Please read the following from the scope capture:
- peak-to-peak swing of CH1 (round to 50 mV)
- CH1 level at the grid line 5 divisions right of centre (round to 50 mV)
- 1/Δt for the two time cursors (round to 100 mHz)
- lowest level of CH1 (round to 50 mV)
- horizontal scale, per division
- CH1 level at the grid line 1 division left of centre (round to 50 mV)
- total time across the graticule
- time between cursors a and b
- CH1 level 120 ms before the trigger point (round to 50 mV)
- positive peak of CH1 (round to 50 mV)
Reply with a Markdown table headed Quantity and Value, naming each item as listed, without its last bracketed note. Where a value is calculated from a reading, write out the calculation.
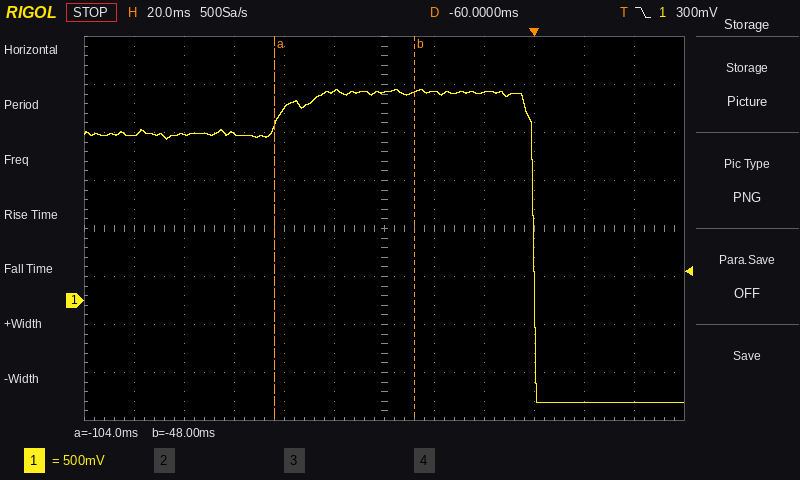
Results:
| Quantity | Value |
|---|---|
| peak-to-peak swing of CH1 | 2.20 V − (-1.05 V) = 3.25 V |
| CH1 level at the grid line 5 divisions right of centre | -1.05 V |
| 1/Δt for the two time cursors | 1 / 56 ms ≈ 17.9 Hz |
| lowest level of CH1 | -1.05 V |
| horizontal scale, per division | 20 ms |
| CH1 level at the grid line 1 division left of centre | 2.20 V |
| total time across the graticule | 240 ms |
| time between cursors a and b | -48 ms − (-104 ms) = 56 ms |
| CH1 level 120 ms before the trigger point | 1.75 V |
| positive peak of CH1 | 2.20 V |
